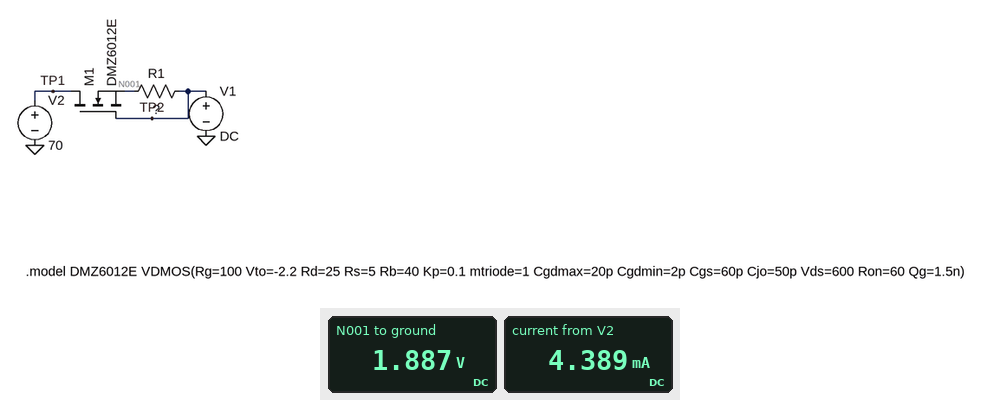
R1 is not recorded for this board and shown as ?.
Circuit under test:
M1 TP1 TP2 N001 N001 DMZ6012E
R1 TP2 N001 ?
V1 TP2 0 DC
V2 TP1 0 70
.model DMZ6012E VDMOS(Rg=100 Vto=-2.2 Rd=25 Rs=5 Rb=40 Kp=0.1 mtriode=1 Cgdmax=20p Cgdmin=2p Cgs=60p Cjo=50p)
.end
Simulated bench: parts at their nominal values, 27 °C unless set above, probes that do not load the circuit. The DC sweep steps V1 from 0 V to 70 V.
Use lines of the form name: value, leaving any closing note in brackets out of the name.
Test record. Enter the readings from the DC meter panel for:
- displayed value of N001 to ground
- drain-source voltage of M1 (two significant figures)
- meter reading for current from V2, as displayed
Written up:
displayed value of N001 to ground: 1.887 V
drain-source voltage of M1: 68 V
meter reading for current from V2, as displayed: 4.389 mA
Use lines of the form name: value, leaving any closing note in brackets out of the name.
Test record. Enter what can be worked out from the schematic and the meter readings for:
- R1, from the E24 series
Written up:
R1, from the E24 series: 430 Ω
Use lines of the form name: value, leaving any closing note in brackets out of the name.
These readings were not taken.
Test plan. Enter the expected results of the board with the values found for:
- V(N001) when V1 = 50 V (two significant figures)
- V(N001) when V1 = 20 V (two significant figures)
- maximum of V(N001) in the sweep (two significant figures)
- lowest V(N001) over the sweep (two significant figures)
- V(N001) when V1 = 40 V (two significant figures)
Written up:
V(N001) when V1 = 50 V: 52 V
V(N001) when V1 = 20 V: 22 V
maximum of V(N001) in the sweep: 70 V
lowest V(N001) over the sweep: 1.9 V
V(N001) when V1 = 40 V: 42 V
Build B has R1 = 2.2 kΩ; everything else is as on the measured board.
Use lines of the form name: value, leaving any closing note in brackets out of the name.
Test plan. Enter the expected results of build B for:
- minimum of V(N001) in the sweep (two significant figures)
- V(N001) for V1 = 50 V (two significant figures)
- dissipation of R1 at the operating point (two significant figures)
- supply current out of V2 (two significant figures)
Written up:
minimum of V(N001) in the sweep: 2.1 V
V(N001) for V1 = 50 V: 52 V
dissipation of R1 at the operating point: 2.0 mW
supply current out of V2: 950 µA
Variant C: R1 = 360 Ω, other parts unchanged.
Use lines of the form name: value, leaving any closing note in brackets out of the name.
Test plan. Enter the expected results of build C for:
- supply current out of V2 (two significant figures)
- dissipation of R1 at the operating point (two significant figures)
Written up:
supply current out of V2: 5.2 mA
dissipation of R1 at the operating point: 9.6 mW
